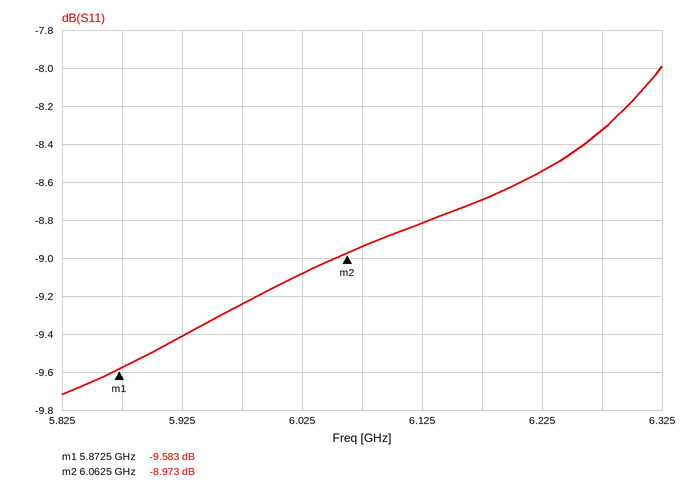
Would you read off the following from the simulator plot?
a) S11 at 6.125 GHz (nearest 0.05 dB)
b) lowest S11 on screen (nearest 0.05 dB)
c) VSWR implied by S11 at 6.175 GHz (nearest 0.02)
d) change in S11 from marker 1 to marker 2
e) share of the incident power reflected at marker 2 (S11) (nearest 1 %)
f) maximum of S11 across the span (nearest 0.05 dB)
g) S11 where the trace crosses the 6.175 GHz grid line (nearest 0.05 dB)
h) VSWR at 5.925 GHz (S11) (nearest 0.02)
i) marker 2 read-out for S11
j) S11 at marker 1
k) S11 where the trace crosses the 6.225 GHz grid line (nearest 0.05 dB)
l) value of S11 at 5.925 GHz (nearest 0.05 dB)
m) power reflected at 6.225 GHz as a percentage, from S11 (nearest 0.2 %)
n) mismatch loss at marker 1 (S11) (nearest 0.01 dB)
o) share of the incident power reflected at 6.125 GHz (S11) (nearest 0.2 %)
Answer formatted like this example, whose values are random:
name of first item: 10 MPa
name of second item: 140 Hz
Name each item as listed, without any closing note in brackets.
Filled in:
S11 at 6.125 GHz: -8.80 dB
lowest S11 on screen: -9.70 dB
VSWR implied by S11 at 6.175 GHz: 2.16
change in S11 from marker 1 to marker 2: 0.610 dB
share of the incident power reflected at marker 2 (S11): 13 %
maximum of S11 across the span: -8.00 dB
S11 where the trace crosses the 6.175 GHz grid line: -8.70 dB
VSWR at 5.925 GHz (S11): 2.02
marker 2 read-out for S11: -8.973 dB
S11 at marker 1: -9.583 dB
S11 where the trace crosses the 6.225 GHz grid line: -8.55 dB
value of S11 at 5.925 GHz: -9.40 dB
power reflected at 6.225 GHz as a percentage, from S11: 14.0 %
mismatch loss at marker 1 (S11): 0.51 dB
share of the incident power reflected at 6.125 GHz (S11): 13.2 %
